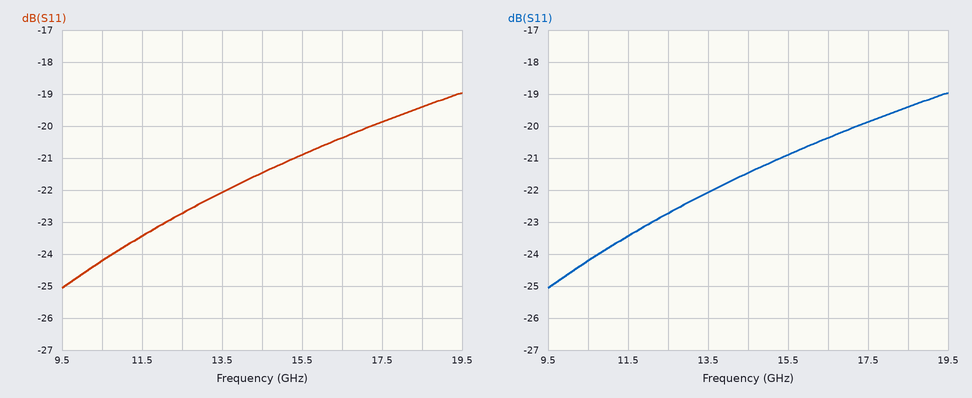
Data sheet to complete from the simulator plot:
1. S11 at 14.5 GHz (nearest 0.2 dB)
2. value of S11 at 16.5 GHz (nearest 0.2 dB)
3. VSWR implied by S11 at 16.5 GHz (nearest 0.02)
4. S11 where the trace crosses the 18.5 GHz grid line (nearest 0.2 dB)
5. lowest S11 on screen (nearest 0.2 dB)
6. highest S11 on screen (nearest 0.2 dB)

-21.4 dB
-20.4 dB
1.22
-19.4 dB
-25.0 dB
-19.0 dB
